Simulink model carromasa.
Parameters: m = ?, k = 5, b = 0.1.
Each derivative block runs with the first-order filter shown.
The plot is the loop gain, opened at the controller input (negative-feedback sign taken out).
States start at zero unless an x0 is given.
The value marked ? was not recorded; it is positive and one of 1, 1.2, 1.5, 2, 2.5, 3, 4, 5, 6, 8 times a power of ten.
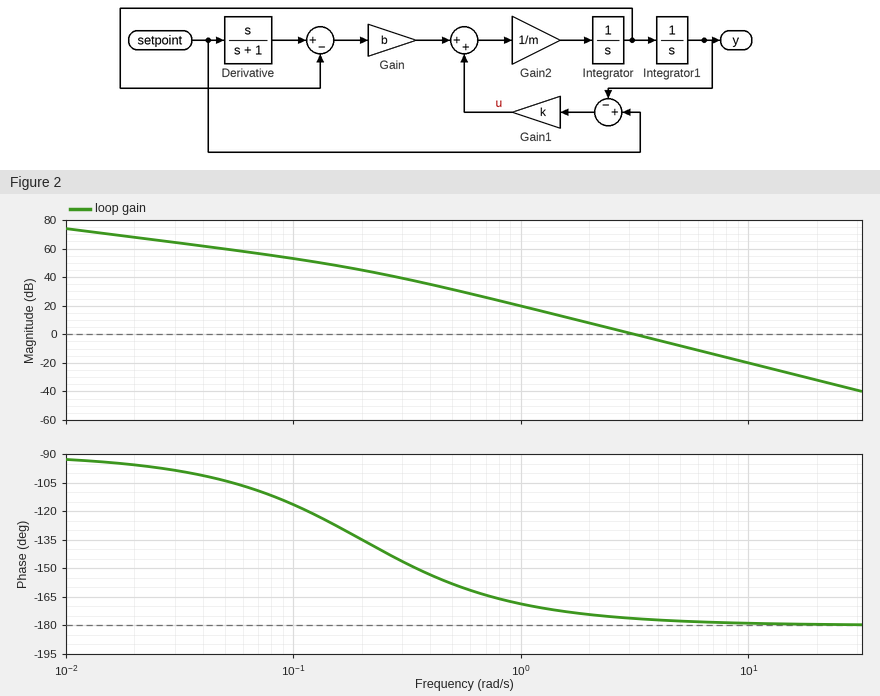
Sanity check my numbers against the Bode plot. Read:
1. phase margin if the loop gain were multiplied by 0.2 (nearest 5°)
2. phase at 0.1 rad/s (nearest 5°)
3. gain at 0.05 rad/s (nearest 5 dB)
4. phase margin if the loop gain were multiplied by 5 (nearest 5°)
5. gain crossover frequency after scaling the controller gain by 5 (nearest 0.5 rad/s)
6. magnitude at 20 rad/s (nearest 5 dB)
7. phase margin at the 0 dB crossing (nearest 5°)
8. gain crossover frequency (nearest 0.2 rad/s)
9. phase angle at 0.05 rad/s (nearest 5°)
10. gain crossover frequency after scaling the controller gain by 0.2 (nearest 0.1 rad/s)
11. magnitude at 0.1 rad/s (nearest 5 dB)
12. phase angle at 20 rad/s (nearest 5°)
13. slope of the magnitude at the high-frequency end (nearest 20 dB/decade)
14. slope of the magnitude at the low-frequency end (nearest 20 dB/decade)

10°
-115°
60 dB
0°
7.0 rad/s
-30 dB
5°
3.2 rad/s
-105°
1.4 rad/s
55 dB
-180°
-40 dB/decade
-20 dB/decade
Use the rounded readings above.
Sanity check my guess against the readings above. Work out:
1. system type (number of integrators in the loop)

1
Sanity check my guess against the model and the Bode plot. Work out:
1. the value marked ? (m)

0.5
